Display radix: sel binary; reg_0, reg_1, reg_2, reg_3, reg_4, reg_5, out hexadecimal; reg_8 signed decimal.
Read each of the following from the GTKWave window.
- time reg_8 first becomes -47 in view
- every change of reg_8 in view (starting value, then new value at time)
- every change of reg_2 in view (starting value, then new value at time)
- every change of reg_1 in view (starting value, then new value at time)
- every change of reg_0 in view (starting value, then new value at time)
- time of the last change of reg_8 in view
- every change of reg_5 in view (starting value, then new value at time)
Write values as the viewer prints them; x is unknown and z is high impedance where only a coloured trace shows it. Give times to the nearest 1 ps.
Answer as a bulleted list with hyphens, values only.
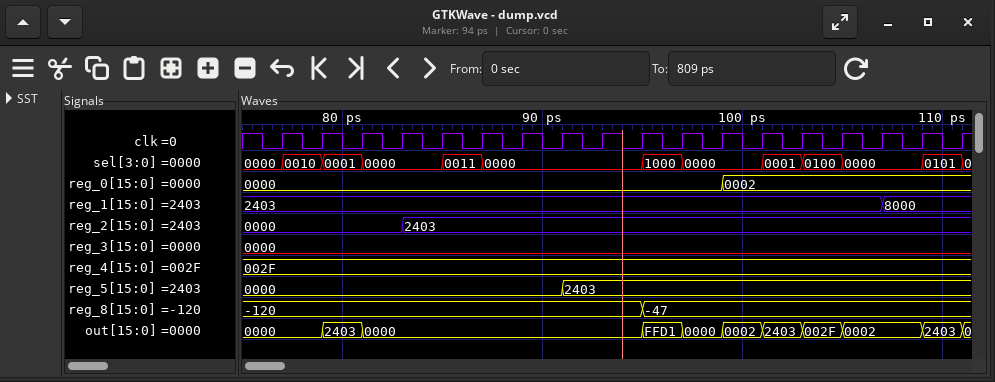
- 95 ps
- -120, -47 at 95 ps
- 0000, 2403 at 83 ps
- 2403, 8000 at 107 ps
- 0000, 0002 at 99 ps
- 95 ps
- 0000, 2403 at 91 ps
